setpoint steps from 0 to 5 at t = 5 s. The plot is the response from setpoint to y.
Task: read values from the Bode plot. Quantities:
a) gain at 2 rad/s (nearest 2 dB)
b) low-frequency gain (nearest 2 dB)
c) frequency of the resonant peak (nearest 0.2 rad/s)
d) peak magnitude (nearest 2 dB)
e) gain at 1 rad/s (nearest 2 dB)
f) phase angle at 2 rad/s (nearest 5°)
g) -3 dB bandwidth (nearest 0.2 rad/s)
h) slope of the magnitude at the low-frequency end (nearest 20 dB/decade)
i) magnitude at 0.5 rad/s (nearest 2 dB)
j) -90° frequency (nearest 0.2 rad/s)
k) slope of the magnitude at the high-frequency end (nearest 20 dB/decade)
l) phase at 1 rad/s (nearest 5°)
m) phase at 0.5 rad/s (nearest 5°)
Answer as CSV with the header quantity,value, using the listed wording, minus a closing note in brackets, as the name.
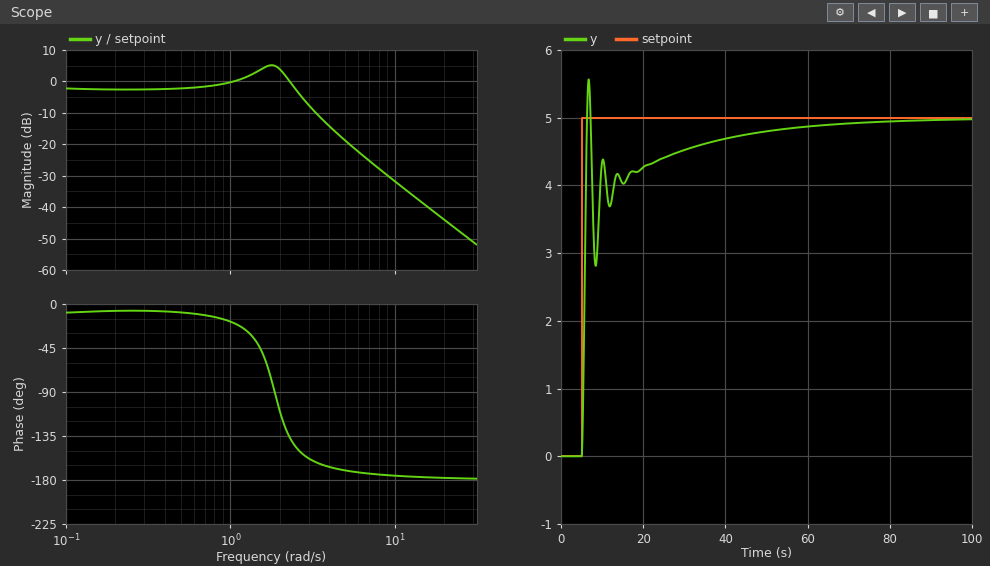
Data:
quantity,value
gain at 2 rad/s,4 dB
low-frequency gain,-2 dB
frequency of the resonant peak,1.8 rad/s
peak magnitude,6 dB
gain at 1 rad/s,0 dB
phase angle at 2 rad/s,-110°
-3 dB bandwidth,2.8 rad/s
slope of the magnitude at the low-frequency end,0 dB/decade
magnitude at 0.5 rad/s,-2 dB
-90° frequency,1.8 rad/s
slope of the magnitude at the high-frequency end,-40 dB/decade
phase at 1 rad/s,-20°
phase at 0.5 rad/s,-10°
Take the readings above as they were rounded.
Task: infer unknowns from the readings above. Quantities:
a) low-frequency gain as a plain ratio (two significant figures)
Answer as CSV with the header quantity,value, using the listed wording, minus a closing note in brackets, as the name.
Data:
quantity,value
low-frequency gain as a plain ratio,0.79
